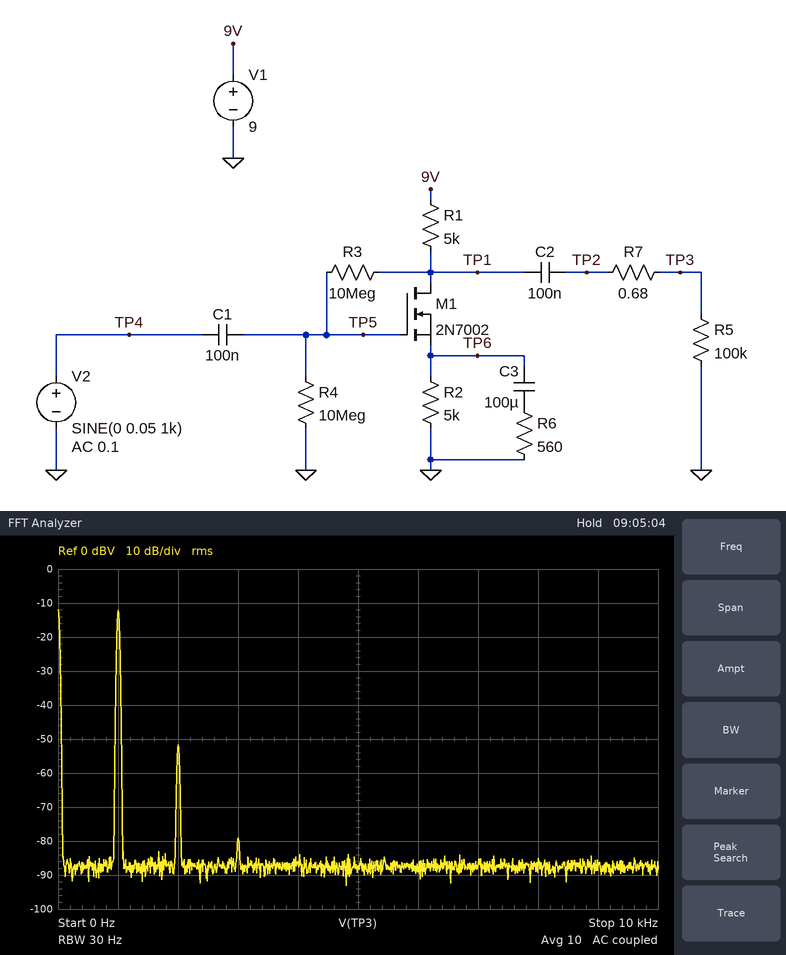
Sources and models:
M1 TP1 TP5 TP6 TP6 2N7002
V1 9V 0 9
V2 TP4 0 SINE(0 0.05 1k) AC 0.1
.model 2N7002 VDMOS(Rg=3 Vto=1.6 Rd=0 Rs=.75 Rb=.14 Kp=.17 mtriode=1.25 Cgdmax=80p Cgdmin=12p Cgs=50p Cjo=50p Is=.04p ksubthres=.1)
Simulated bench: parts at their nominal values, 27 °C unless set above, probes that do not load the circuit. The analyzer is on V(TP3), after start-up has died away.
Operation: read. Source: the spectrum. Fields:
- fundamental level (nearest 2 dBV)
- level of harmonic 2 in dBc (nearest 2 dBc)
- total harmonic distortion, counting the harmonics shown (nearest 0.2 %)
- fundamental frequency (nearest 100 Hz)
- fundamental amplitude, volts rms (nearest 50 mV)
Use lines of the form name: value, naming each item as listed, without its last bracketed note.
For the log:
fundamental level: -12 dBV
level of harmonic 2 in dBc: -40 dBc
total harmonic distortion, counting the harmonics shown: 1.0 %
fundamental frequency: 1.0 kHz
fundamental amplitude, volts rms: 250 mV
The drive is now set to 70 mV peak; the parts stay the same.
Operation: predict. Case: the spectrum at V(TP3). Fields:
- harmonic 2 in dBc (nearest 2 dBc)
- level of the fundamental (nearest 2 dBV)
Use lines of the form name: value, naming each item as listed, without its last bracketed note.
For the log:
harmonic 2 in dBc: -36 dBc
level of the fundamental: -10 dBV
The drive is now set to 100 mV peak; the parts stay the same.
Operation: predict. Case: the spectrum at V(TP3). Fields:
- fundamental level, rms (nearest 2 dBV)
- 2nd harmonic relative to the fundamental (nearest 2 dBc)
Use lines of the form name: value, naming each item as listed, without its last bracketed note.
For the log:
fundamental level, rms: -6 dBV
2nd harmonic relative to the fundamental: -34 dBc
